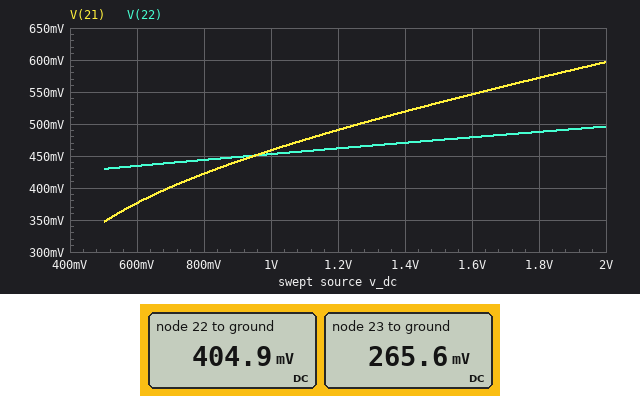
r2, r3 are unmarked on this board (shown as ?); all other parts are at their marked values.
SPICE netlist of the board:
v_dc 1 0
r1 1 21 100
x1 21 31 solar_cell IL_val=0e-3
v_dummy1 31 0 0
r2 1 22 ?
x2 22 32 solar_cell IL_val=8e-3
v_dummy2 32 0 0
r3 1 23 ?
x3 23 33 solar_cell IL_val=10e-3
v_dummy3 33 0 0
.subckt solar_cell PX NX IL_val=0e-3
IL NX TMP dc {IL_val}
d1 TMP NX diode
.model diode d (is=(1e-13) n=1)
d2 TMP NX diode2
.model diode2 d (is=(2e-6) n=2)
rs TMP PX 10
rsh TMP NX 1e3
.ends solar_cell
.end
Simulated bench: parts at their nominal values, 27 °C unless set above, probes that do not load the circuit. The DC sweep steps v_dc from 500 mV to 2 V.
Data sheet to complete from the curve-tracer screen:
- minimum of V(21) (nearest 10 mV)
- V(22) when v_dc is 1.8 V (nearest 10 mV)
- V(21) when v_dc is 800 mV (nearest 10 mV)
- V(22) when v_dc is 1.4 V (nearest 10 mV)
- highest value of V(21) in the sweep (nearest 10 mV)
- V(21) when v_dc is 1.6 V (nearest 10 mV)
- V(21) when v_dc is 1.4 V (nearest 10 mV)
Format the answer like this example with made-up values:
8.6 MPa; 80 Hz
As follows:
350 mV; 490 mV; 420 mV; 470 mV; 600 mV; 550 mV; 520 mV
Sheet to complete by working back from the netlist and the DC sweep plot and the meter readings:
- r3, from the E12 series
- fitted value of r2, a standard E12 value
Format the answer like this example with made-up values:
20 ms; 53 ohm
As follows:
33 Ω; 330 Ω
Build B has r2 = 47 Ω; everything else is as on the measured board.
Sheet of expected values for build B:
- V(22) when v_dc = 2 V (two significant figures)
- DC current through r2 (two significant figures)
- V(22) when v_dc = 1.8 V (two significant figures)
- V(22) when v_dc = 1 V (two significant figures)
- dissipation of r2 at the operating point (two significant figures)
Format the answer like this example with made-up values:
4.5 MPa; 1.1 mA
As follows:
770 mV; 6.1 mA; 730 mV; 560 mV; 1.7 mW
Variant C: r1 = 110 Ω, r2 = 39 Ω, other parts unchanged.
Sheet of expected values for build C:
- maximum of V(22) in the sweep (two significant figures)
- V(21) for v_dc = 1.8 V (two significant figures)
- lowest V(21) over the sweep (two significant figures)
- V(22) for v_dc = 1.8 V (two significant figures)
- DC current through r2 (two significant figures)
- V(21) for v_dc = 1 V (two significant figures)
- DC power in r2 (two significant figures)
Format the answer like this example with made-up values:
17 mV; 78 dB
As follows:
810 mV; 560 mV; 340 mV; 770 mV; 6.6 mA; 450 mV; 1.7 mW
